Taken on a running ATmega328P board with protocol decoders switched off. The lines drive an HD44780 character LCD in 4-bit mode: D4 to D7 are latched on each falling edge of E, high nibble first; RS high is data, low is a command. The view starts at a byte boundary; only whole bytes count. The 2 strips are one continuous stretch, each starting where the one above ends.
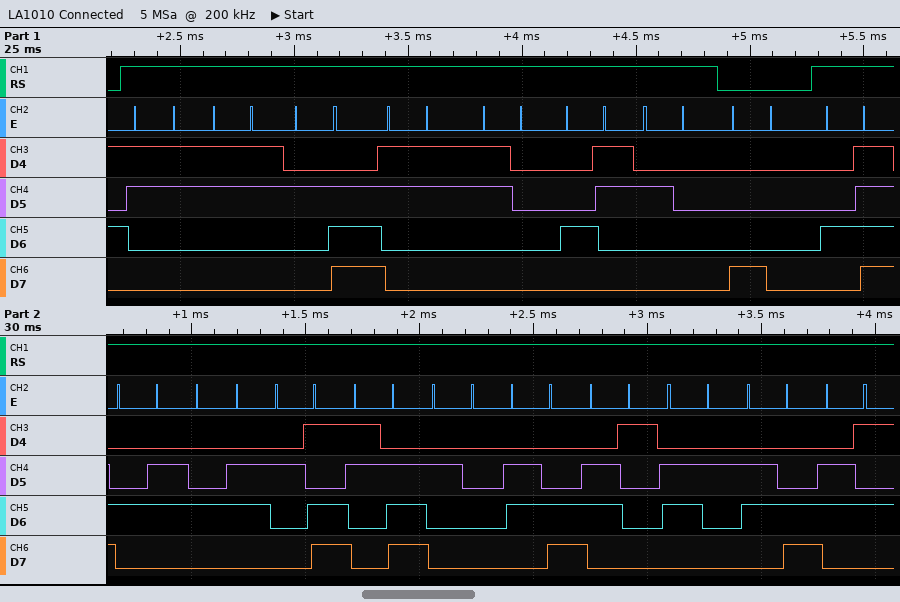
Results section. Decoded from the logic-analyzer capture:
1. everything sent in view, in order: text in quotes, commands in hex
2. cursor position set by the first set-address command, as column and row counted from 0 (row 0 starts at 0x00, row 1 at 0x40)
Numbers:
"33.30C " 0x80 "OFF-> lable"
column 0, row 0
